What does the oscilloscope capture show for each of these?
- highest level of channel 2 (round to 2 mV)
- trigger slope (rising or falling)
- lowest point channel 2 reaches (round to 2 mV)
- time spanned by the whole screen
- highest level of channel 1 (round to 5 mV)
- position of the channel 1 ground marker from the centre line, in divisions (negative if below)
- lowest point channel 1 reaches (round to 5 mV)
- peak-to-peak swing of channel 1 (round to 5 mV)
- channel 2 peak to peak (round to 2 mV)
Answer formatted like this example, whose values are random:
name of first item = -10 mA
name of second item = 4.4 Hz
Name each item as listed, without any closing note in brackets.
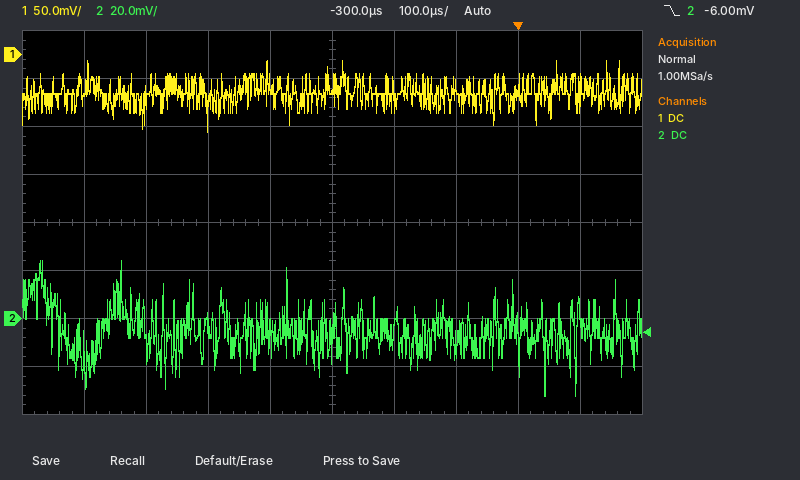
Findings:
highest level of channel 2 = 24 mV
trigger slope = falling
lowest point channel 2 reaches = -32 mV
time spanned by the whole screen = 1 ms
highest level of channel 1 = -5 mV
position of the channel 1 ground marker from the centre line, in divisions = +3.5 div
lowest point channel 1 reaches = -80 mV
peak-to-peak swing of channel 1 = 75 mV
channel 2 peak to peak = 56 mV
